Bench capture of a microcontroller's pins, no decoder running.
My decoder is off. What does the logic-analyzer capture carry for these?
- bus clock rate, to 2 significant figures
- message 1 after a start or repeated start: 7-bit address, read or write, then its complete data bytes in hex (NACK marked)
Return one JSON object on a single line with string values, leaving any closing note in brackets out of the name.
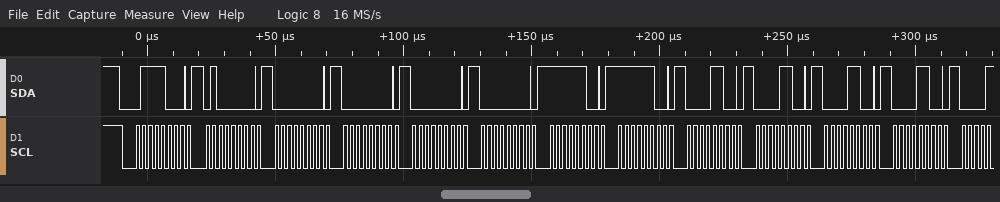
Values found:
{"bus clock rate, to 2 significant figures": "400 kHz", "message 1 after a start or repeated start: 7-bit address, read or write, then its complete data bytes in hex": "0x3C write: 40 00 00 00 00 FC FC 0C 0C 0C 0C"}
